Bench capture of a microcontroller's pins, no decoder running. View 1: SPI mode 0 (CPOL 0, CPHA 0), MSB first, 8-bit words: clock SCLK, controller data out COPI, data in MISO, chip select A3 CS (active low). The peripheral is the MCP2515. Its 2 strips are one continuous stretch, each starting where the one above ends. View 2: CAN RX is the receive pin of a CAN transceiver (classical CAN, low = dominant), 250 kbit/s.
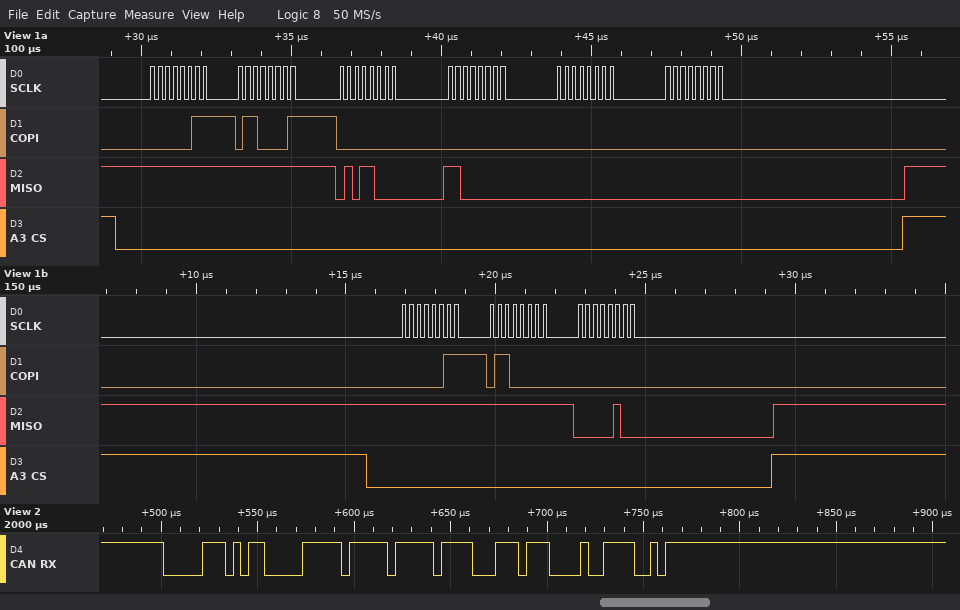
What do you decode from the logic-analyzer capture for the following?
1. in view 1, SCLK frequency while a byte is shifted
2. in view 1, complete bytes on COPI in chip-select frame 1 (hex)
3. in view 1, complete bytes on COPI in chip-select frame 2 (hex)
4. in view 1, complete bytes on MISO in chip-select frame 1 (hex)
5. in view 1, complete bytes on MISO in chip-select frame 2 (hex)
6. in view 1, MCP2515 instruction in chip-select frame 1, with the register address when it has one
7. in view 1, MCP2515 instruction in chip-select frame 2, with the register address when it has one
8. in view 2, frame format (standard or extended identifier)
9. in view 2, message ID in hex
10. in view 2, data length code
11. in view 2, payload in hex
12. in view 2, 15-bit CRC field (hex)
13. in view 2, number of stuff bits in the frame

4 MHz
0x03 0x61 0x00 0x00 0x00 0x00
0x03 0x60 0x00
0xFF 0xFF 0x58 0xC0 0x00 0x00
0xFF 0xFF 0x04
READ 0x61
READ 0x60
standard
0x06B
3
FF FF 1D
0x613C
5
